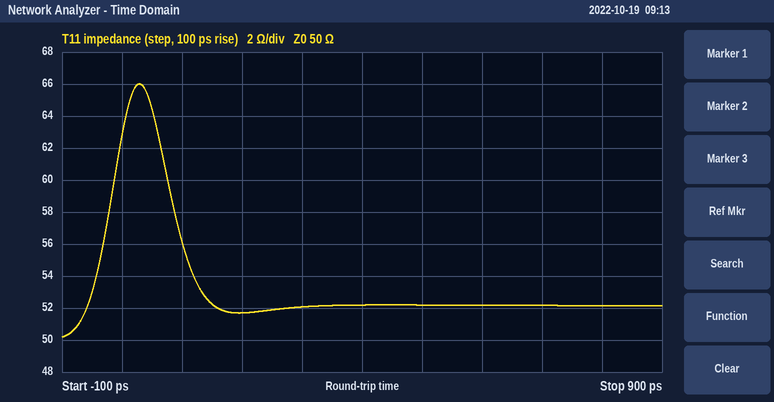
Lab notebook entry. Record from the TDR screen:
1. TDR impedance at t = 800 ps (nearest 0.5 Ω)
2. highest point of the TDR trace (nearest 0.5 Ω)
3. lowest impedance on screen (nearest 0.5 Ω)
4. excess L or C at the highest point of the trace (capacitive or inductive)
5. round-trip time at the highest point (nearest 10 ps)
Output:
52.0 Ω
66.0 Ω
50.0 Ω
inductive
30 ps
